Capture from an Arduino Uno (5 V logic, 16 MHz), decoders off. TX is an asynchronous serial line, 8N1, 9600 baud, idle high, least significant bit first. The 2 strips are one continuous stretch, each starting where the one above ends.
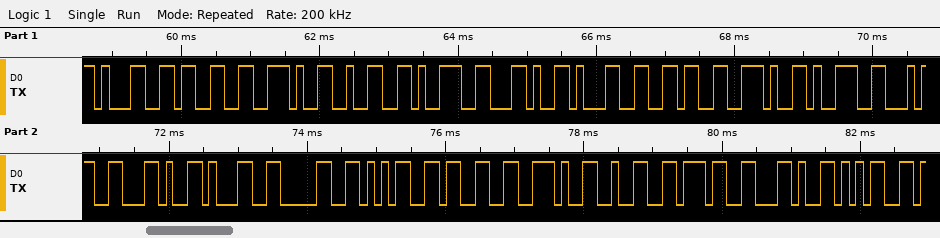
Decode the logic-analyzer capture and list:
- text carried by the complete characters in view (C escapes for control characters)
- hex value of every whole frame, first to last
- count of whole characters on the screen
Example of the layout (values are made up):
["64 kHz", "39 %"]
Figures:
["\"13.29,16.94,1053.27,5\"", "31 33 2E 32 39 2C 31 36 2E 39 34 2C 31 30 35 33 2E 32 37 2C 35", "21"]
